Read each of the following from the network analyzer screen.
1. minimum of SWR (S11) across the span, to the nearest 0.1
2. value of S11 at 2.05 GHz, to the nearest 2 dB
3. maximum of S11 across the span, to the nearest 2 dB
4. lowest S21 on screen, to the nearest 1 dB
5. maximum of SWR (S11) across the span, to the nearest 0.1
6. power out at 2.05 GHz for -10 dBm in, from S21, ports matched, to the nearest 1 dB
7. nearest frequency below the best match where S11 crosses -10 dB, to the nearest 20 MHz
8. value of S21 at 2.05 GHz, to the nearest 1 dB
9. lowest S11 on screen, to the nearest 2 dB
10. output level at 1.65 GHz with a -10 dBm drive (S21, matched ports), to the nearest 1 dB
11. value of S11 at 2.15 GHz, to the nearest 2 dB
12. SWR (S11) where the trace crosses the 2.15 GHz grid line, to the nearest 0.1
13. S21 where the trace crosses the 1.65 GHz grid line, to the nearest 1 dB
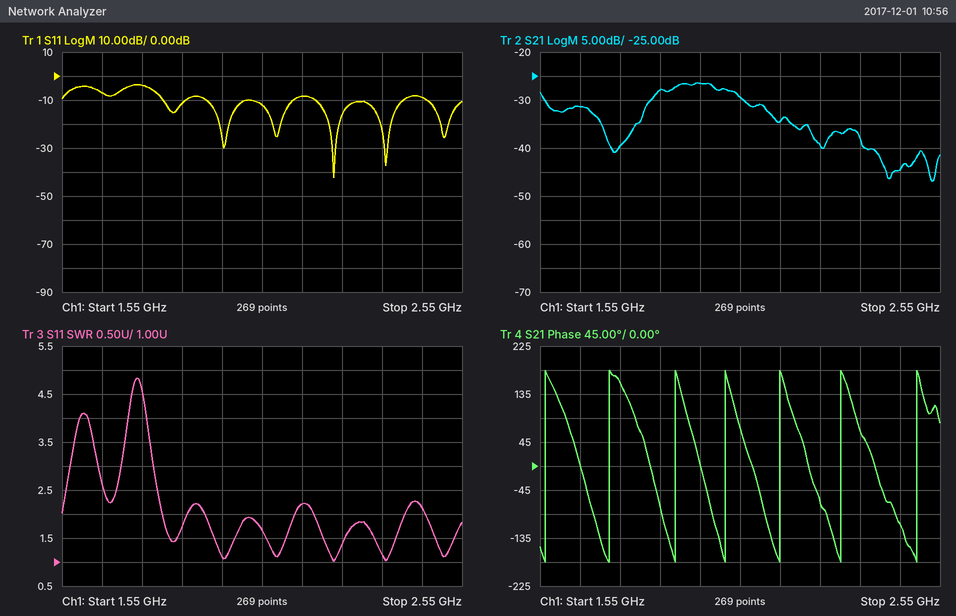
1.0
-12 dB
-4 dB
-47 dB
4.8
-39 dBm
2.18 GHz
-29 dB
-42 dB
-41 dBm
-8 dB
2.2
-31 dB
